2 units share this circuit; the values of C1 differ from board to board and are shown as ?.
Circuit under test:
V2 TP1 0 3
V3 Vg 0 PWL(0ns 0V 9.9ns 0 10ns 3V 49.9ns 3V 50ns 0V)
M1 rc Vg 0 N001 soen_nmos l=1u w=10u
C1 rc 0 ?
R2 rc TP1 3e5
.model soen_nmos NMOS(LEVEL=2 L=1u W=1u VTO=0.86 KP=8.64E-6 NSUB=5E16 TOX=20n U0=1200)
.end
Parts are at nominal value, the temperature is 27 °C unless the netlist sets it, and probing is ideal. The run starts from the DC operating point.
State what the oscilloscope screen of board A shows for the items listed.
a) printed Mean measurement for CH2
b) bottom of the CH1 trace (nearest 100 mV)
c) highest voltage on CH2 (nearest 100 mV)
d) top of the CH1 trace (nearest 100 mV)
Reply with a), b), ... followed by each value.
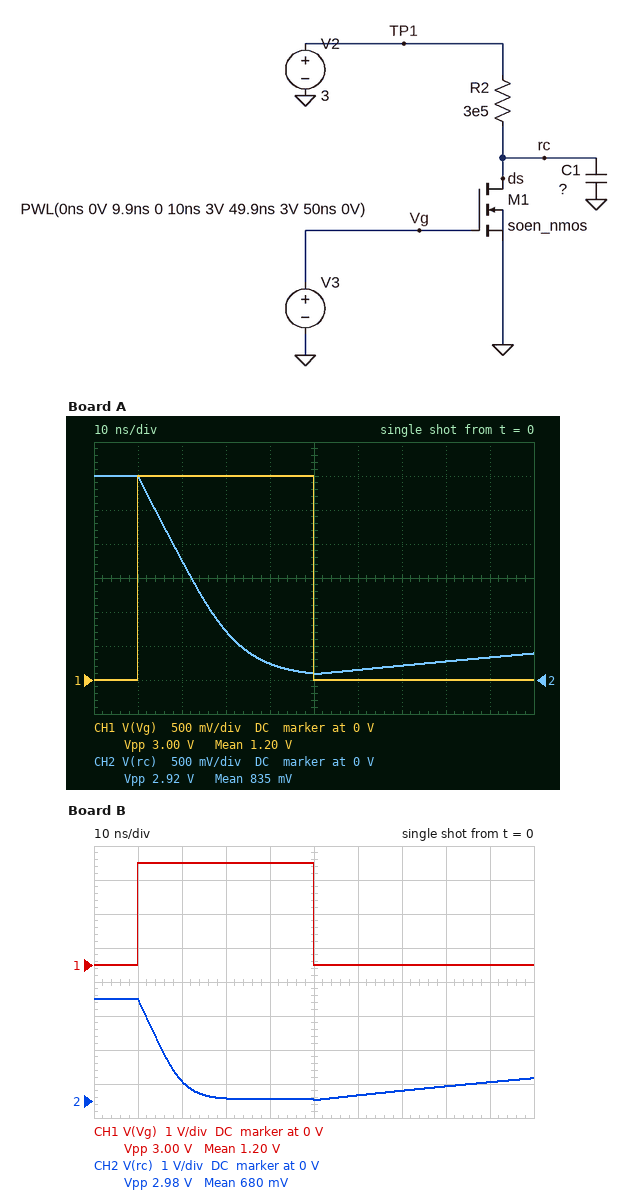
a) 835 mV
b) 0 V
c) 3.0 V
d) 3.0 V
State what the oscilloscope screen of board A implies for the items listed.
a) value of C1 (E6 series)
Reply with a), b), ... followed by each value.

a) 1.5 pF
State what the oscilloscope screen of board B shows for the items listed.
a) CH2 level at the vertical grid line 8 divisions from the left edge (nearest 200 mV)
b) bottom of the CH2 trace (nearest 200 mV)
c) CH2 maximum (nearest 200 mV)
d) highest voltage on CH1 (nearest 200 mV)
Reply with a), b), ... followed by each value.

a) 400 mV
b) 0 V
c) 3.0 V
d) 3.0 V
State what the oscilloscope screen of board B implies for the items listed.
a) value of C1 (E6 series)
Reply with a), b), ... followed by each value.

a) 680 fF
